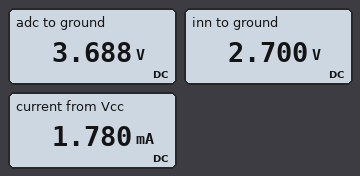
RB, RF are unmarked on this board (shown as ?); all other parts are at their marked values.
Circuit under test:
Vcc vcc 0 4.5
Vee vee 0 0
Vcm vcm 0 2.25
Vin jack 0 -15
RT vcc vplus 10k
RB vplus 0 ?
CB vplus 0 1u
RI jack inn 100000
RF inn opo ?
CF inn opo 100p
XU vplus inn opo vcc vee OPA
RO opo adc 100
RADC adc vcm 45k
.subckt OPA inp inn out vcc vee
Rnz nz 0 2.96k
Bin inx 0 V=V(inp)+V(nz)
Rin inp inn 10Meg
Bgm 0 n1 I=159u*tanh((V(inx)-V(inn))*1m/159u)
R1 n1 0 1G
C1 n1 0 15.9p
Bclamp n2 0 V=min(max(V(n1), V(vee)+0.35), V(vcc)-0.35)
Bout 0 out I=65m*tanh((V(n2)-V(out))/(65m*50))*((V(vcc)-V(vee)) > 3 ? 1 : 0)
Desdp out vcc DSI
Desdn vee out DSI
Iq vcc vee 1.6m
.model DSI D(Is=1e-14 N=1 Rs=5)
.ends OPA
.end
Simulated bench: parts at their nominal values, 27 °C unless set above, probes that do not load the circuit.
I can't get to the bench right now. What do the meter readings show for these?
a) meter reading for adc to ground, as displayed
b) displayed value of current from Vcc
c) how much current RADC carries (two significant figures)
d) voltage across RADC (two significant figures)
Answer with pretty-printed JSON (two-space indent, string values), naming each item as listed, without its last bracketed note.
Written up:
{
  "meter reading for adc to ground, as displayed": "3.688 V",
  "displayed value of current from Vcc": "1.780 mA",
  "how much current RADC carries": "32 µA",
  "voltage across RADC": "1.4 V"
}
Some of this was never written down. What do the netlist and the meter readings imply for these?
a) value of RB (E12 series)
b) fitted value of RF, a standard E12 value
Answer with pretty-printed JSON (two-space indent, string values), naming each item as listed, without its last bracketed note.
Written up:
{
  "value of RB": "15 kΩ",
  "fitted value of RF, a standard E12 value": "5.6 kΩ"
}
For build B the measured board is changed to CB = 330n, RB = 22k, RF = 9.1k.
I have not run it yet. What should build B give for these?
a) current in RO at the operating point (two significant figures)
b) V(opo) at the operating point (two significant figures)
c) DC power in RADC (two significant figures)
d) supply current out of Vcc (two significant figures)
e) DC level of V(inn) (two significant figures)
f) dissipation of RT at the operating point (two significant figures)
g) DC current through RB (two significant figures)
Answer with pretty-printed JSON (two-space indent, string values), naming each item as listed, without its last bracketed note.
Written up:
{
  "current in RO at the operating point": "42 µA",
  "V(opo) at the operating point": "4.1 V",
  "DC power in RADC": "79 µW",
  "supply current out of Vcc": "1.7 mA",
  "DC level of V(inn)": "2.5 V",
  "dissipation of RT at the operating point": "200 µW",
  "DC current through RB": "140 µA"
}
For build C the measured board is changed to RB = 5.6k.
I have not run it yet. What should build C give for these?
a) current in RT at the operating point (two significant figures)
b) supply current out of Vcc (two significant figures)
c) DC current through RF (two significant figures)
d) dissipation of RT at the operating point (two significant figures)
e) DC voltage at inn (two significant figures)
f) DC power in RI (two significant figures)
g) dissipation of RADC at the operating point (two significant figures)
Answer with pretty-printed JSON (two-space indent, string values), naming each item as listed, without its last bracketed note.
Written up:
{
  "current in RT at the operating point": "290 µA",
  "supply current out of Vcc": "1.9 mA",
  "DC current through RF": "170 µA",
  "dissipation of RT at the operating point": "830 µW",
  "DC voltage at inn": "1.6 V",
  "DC power in RI": "2.8 mW",
  "dissipation of RADC at the operating point": "1.9 µW"
}
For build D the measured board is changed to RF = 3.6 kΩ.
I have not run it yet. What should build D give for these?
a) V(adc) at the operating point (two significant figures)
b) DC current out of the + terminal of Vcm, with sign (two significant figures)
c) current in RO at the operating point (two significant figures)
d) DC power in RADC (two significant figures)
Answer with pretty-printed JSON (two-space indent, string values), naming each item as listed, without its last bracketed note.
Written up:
{
  "V(adc) at the operating point": "3.3 V",
  "DC current out of the + terminal of Vcm, with sign": "-24 µA",
  "current in RO at the operating point": "24 µA",
  "DC power in RADC": "26 µW"
}
